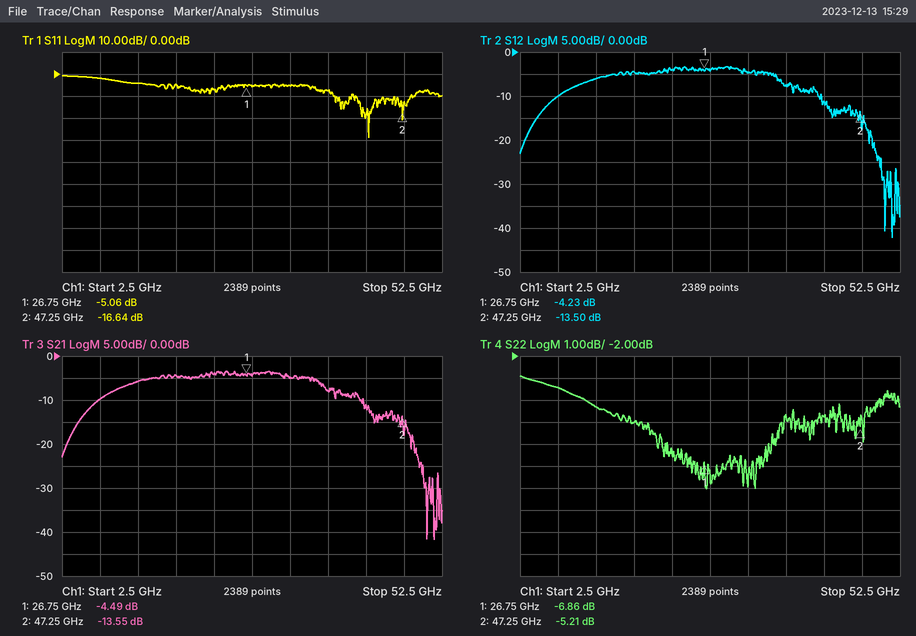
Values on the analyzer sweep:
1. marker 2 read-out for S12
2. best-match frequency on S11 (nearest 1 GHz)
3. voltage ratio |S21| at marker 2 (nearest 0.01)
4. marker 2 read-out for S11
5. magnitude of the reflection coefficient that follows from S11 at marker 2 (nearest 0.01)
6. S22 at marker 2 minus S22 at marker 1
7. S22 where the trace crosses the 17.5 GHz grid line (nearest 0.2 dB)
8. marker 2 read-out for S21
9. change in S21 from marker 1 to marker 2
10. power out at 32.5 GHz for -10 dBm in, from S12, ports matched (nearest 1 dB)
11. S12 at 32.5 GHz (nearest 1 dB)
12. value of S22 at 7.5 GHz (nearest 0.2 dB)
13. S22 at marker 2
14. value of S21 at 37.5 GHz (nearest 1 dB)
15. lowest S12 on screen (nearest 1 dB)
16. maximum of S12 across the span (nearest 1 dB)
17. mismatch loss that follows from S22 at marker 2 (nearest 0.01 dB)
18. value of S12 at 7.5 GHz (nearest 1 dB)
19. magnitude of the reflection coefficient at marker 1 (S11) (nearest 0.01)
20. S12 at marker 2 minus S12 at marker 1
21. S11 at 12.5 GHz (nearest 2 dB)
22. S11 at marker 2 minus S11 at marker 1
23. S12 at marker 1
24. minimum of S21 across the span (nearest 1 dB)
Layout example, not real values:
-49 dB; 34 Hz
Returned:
-13.50 dB; 43 GHz; 0.21; -16.64 dB; 0.15; 1.65 dB; -5.0 dB; -13.55 dB; -9.06 dB; -15 dBm; -5 dB; -3.4 dB; -5.21 dB; -8 dB; -42 dB; -3 dB; 1.56 dB; -10 dB; 0.56; -9.27 dB; -4 dB; -11.58 dB; -4.23 dB; -42 dB
